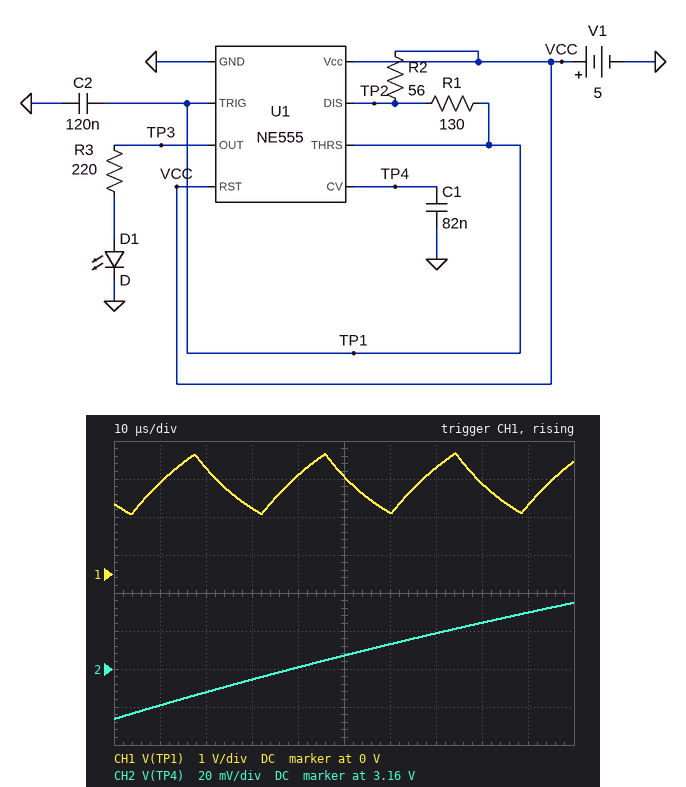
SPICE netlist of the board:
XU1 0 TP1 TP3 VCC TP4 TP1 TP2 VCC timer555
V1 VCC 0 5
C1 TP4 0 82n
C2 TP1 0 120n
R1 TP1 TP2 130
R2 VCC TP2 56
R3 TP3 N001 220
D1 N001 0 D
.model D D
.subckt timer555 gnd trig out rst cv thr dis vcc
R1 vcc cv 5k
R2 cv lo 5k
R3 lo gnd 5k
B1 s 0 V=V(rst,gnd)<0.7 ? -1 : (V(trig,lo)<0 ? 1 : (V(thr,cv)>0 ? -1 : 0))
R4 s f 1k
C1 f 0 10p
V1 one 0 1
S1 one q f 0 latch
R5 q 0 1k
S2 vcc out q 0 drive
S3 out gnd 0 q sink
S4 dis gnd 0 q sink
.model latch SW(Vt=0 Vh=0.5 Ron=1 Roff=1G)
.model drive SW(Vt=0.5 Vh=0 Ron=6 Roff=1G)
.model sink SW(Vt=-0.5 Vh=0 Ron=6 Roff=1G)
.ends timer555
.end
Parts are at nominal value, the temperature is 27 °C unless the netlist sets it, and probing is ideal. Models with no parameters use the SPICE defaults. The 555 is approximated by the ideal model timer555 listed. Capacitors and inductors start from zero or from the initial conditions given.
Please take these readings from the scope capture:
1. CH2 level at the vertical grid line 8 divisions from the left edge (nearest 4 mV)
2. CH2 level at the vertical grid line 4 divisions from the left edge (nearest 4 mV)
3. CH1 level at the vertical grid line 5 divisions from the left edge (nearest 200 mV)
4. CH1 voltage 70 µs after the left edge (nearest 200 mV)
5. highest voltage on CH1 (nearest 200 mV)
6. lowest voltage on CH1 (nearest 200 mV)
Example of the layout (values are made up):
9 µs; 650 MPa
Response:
3.184 V; 3.160 V; 2.6 V; 2.8 V; 3.2 V; 1.6 V
